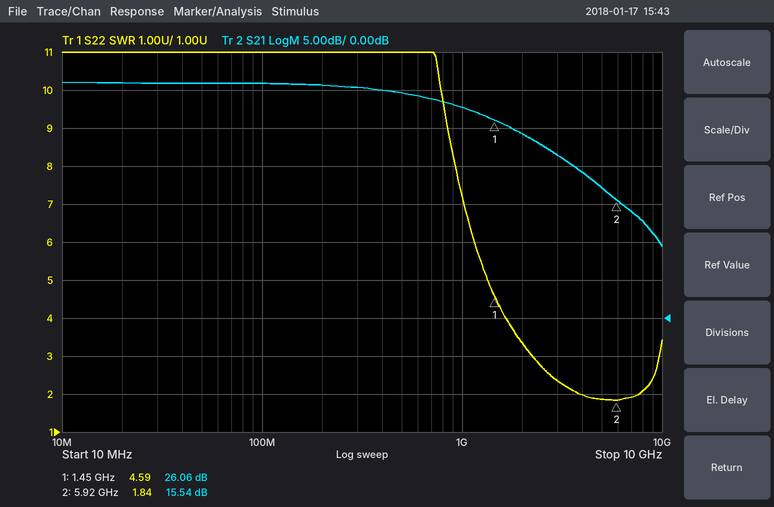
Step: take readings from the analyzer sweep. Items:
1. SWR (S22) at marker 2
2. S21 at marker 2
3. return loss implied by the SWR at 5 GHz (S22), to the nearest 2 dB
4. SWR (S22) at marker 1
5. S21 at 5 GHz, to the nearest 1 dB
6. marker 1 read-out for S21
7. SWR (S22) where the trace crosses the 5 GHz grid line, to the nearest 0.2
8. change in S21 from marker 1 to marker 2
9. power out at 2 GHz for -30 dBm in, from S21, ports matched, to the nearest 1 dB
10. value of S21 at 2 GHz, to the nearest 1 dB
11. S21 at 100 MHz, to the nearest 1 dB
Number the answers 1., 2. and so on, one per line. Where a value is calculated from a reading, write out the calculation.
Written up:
1. 1.84
2. 15.54 dB
3. −20 log10((1.8 − 1)/(1.8 + 1)) ≈ 10.9 dB, so 10 dB to the nearest 2 dB
4. 4.59
5. 17 dB
6. 26.06 dB
7. 1.8
8. 15.54 − (26.06) = -10.52 dB
9. -30 dBm + (24 dB) = -6 dBm
10. 24 dB
11. 31 dB
